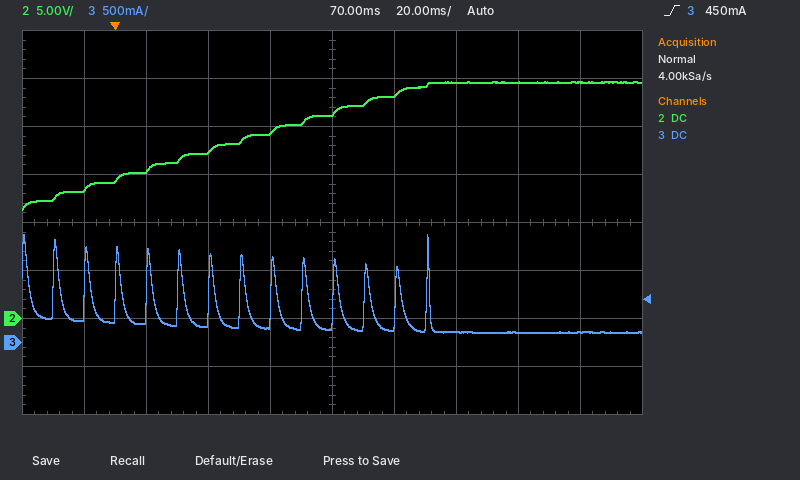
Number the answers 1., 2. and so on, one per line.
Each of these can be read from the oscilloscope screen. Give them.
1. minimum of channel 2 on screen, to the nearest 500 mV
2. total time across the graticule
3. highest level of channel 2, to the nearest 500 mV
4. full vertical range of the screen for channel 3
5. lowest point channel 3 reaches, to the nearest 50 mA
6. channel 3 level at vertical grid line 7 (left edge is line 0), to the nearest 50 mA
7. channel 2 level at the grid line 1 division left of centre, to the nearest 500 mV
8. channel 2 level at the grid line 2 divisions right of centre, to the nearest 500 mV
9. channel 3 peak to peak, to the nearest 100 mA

1. 11.5 V
2. 200 ms
3. 24.5 V
4. 4 A
5. 100 mA
6. 100 mA
7. 19.5 V
8. 24.5 V
9. 1.00 A
